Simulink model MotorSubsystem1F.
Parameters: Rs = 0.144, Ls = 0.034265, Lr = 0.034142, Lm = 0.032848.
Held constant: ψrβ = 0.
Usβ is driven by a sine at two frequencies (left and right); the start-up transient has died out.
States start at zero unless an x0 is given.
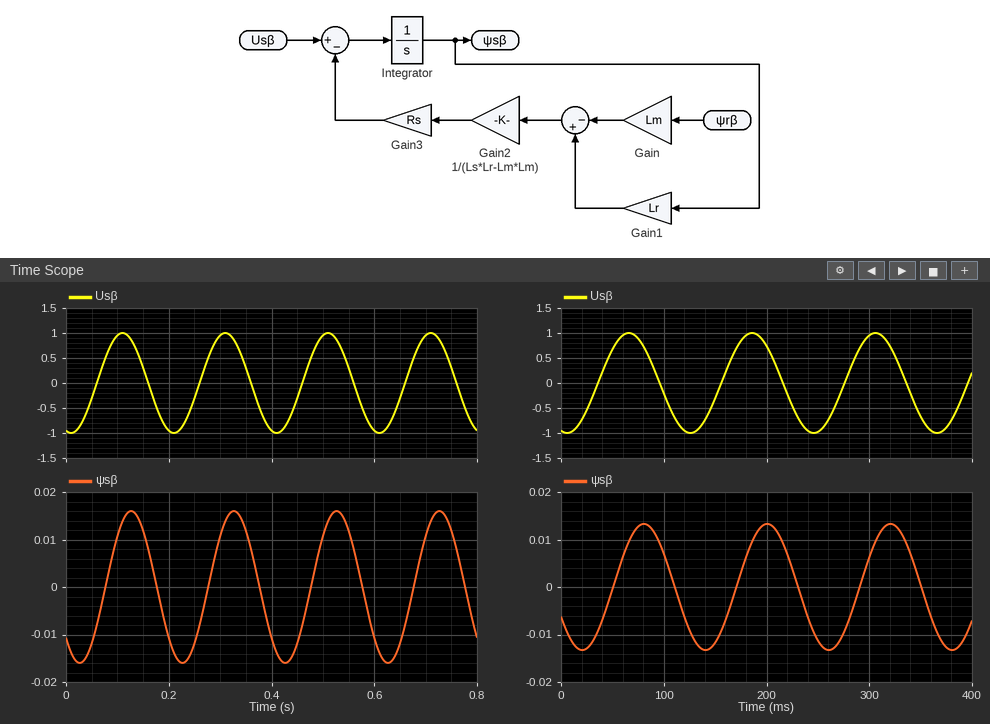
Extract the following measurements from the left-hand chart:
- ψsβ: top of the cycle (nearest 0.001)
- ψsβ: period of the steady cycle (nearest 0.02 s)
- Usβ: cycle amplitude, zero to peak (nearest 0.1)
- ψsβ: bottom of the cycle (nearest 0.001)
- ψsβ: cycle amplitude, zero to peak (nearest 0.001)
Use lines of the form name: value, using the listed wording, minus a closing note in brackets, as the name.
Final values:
ψsβ: top of the cycle: 0.016
ψsβ: period of the steady cycle: 0.20 s
Usβ: cycle amplitude, zero to peak: 1.0
ψsβ: bottom of the cycle: -0.016
ψsβ: cycle amplitude, zero to peak: 0.016
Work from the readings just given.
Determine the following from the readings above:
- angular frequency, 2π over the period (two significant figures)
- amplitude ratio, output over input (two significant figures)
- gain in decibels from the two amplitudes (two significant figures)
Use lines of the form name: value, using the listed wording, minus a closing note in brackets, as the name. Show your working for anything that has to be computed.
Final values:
angular frequency, 2π over the period: 2π / 0.2 = 31 rad/s
amplitude ratio, output over input: 0.016 / 1 = 0.016
gain in decibels from the two amplitudes: 20 log10(0.016 / 1) = -36 dB
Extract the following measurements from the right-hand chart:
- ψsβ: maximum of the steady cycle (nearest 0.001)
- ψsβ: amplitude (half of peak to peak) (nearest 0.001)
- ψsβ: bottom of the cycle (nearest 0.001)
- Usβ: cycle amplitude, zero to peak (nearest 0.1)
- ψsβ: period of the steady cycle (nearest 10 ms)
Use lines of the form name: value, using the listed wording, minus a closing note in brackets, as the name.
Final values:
ψsβ: maximum of the steady cycle: 0.013
ψsβ: amplitude (half of peak to peak): 0.013
ψsβ: bottom of the cycle: -0.013
Usβ: cycle amplitude, zero to peak: 1.0
ψsβ: period of the steady cycle: 120 ms
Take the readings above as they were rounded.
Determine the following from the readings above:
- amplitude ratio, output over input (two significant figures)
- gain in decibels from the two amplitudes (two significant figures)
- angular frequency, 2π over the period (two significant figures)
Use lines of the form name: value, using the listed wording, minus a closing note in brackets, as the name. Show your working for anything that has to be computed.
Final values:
amplitude ratio, output over input: 0.013 / 1 = 0.013
gain in decibels from the two amplitudes: 20 log10(0.013 / 1) = -38 dB
angular frequency, 2π over the period: 2π / 120 = 0.052 rad/ms
